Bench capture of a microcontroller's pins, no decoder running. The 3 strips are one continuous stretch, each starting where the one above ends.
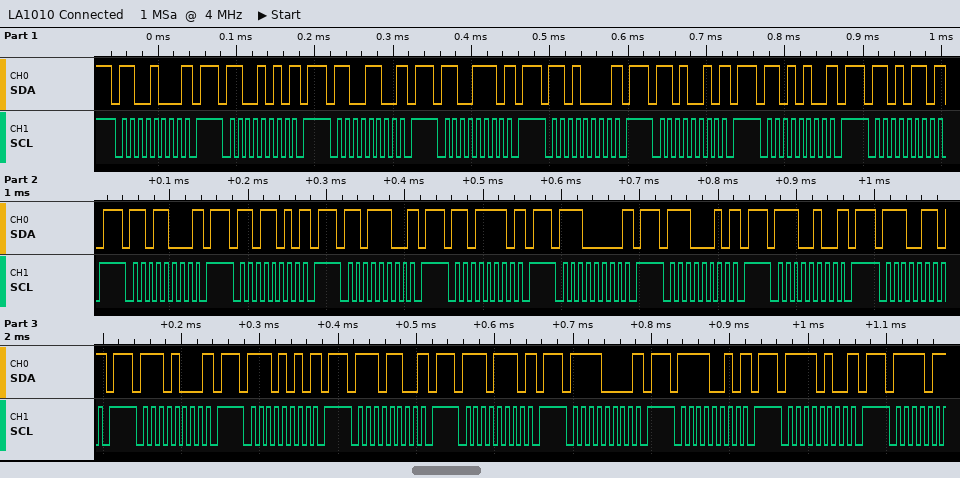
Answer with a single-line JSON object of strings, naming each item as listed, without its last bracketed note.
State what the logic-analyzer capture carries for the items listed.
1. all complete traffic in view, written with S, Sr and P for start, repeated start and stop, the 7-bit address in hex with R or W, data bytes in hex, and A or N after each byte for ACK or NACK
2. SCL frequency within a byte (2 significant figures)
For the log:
{"all complete traffic in view, written with S, Sr and P for start, repeated start and stop, the 7-bit address in hex with R or W, data bytes in hex, and A or N after each byte for ACK or NACK": "S 64W N P S 65W N P S 66W N P S 67W N P S 68W N P S 69W N P S 6AW N P S 6BW N P S 6CW N P S 6DW N P S 6EW N P S 6FW N P S 70W N P S 71W N P S 72W N P S 73W N P S 74W N P S 75W N P S 76W N P S 77W N P S 78W N P S 79W N P S 7AW N P", "SCL frequency within a byte": "100 kHz"}
